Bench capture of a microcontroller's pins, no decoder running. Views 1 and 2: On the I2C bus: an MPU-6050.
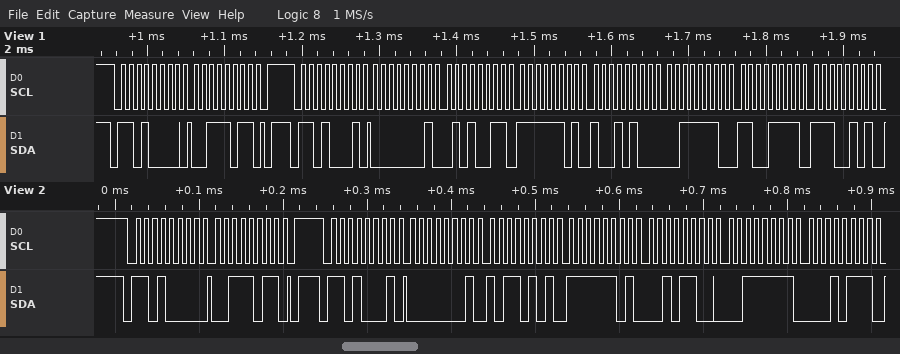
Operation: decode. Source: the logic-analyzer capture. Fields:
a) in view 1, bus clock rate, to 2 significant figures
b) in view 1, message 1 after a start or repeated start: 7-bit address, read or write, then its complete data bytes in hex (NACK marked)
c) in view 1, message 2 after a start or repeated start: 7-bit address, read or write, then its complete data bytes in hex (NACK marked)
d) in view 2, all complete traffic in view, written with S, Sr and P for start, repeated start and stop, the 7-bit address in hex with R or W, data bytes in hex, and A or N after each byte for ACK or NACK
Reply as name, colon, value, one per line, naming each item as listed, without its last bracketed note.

in view 1, bus clock rate, to 2 significant figures: 100 kHz
in view 1, message 1 after a start or repeated start: 7-bit address, read or write, then its complete data bytes in hex: 0x68 write: 3B
in view 1, message 2 after a start or repeated start: 7-bit address, read or write, then its complete data bytes in hex: 0x68 read: 01 53 FD 94 3E CF E5
in view 2, all complete traffic in view, written with S, Sr and P for start, repeated start and stop, the 7-bit address in hex with R or W, data bytes in hex, and A or N after each byte for ACK or NACK: S 68W A 3B A P S 68R A 01 A B5 A FD A 2C A 3F A 17 A
